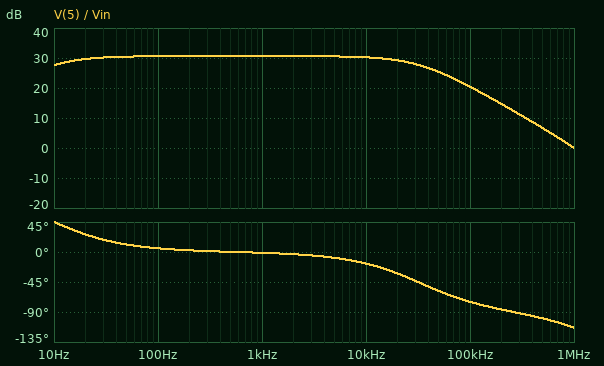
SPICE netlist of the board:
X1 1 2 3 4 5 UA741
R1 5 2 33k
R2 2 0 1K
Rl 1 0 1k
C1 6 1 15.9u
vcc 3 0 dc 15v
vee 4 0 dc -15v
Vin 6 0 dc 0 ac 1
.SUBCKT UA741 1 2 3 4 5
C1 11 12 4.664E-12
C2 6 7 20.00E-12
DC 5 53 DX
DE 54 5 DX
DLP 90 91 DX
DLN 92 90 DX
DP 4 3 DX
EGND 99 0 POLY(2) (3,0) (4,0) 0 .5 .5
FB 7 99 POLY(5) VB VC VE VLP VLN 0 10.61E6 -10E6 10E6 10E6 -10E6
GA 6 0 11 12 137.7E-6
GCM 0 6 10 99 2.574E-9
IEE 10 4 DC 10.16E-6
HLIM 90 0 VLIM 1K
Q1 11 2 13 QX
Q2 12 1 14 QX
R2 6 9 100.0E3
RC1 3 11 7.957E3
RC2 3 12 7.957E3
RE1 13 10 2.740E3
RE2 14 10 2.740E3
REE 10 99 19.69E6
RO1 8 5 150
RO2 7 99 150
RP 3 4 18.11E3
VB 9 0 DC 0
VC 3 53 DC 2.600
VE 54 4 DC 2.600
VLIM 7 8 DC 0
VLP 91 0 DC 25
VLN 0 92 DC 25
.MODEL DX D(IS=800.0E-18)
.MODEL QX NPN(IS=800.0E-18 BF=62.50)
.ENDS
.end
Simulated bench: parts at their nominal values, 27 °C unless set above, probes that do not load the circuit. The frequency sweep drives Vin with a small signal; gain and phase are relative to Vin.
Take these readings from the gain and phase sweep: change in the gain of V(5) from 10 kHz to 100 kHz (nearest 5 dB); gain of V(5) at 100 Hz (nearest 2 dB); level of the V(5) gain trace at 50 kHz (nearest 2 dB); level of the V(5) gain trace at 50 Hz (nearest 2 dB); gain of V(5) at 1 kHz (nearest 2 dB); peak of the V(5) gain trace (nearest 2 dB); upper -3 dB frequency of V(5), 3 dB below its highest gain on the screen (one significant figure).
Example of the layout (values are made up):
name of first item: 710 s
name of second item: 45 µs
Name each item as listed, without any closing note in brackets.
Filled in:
change in the gain of V(5) from 10 kHz to 100 kHz: -10 dB
gain of V(5) at 100 Hz: 30 dB
level of the V(5) gain trace at 50 kHz: 26 dB
level of the V(5) gain trace at 50 Hz: 30 dB
gain of V(5) at 1 kHz: 30 dB
peak of the V(5) gain trace: 30 dB
upper -3 dB frequency of V(5), 3 dB below its highest gain on the screen: 30 kHz
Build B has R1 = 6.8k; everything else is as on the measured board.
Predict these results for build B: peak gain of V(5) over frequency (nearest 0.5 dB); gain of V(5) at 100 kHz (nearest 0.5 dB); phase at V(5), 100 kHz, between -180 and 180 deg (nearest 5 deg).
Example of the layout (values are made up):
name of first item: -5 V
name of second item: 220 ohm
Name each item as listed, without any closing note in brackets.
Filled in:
peak gain of V(5) over frequency: 18.0 dB
gain of V(5) at 100 kHz: 16.0 dB
phase at V(5), 100 kHz, between -180 and 180 deg: -35 deg
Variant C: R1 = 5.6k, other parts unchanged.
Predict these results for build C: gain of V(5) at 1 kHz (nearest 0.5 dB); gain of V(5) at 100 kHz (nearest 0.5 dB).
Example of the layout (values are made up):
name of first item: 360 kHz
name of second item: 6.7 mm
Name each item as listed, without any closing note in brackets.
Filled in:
gain of V(5) at 1 kHz: 16.5 dB
gain of V(5) at 100 kHz: 15.0 dB
